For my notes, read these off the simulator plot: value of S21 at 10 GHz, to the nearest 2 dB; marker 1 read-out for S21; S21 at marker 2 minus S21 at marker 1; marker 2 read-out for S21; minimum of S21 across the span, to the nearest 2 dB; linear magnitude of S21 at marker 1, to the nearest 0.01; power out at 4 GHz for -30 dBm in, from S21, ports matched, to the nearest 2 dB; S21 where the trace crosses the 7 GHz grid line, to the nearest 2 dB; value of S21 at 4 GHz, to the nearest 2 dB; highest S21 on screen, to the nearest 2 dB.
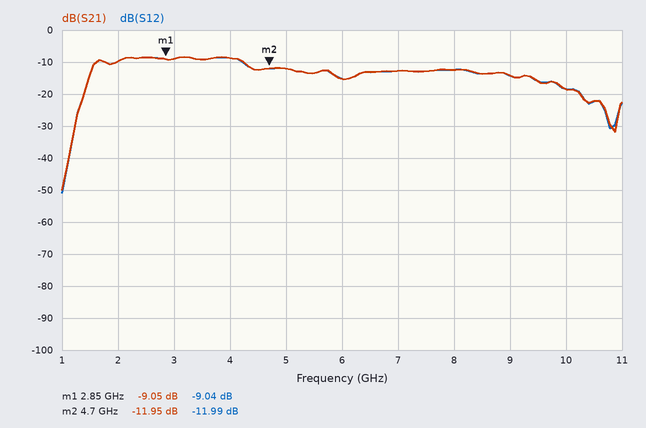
-18 dB
-9.05 dB
-2.90 dB
-11.95 dB
-50 dB
0.35
-38 dBm
-12 dB
-8 dB
-8 dB
